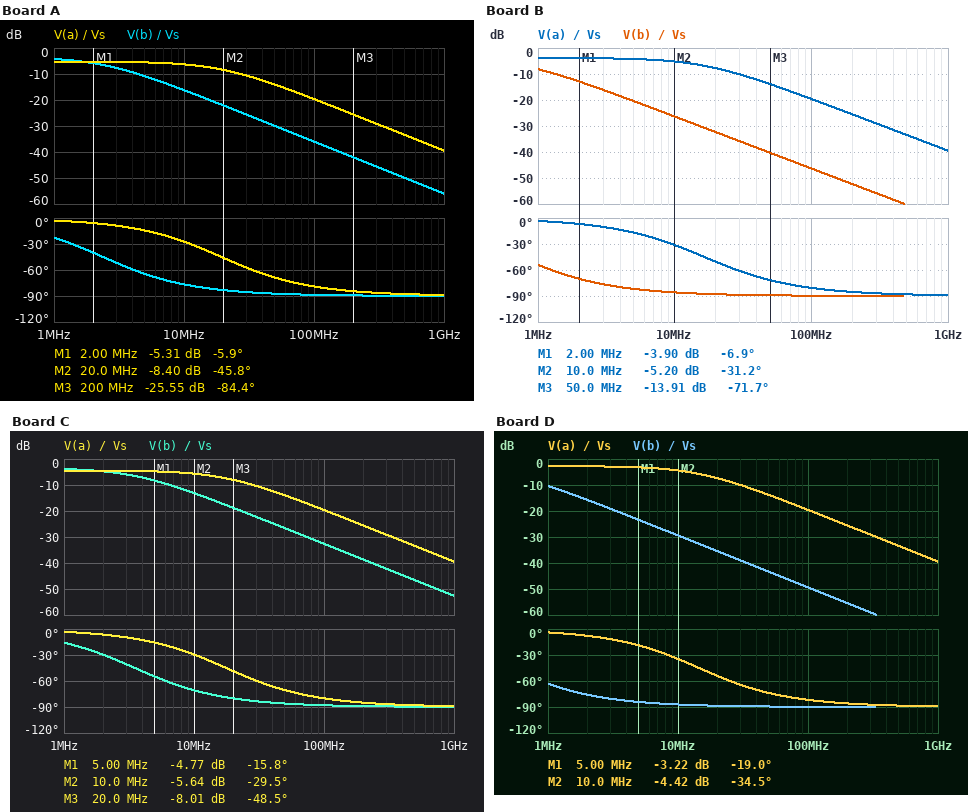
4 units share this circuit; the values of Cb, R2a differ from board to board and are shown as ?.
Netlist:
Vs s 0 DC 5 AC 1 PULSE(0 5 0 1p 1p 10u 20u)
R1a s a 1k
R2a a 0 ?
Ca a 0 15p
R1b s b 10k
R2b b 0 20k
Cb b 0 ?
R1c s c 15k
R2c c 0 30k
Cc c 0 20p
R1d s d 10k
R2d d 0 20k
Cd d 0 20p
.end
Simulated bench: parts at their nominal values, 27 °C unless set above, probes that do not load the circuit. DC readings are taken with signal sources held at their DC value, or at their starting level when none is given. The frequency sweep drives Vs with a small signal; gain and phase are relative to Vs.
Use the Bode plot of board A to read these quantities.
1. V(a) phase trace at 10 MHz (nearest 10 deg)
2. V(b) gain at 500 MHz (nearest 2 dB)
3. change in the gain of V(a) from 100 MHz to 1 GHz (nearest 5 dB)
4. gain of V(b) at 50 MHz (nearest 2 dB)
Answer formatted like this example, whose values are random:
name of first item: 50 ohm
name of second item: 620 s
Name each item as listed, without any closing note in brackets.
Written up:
V(a) phase trace at 10 MHz: -30 deg
V(b) gain at 500 MHz: -50 dB
change in the gain of V(a) from 100 MHz to 1 GHz: -20 dB
gain of V(b) at 50 MHz: -30 dB
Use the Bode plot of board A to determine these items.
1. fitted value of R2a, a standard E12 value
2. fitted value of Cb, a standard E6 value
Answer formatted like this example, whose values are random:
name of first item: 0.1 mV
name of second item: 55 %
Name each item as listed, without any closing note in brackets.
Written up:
fitted value of R2a, a standard E12 value: 1.2 kΩ
fitted value of Cb, a standard E6 value: 10 pF
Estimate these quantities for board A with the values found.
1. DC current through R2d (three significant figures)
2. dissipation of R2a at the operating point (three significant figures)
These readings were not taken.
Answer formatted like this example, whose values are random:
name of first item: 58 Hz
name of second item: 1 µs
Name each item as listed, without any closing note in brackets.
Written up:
DC current through R2d: 167 µA
dissipation of R2a at the operating point: 6.20 mW
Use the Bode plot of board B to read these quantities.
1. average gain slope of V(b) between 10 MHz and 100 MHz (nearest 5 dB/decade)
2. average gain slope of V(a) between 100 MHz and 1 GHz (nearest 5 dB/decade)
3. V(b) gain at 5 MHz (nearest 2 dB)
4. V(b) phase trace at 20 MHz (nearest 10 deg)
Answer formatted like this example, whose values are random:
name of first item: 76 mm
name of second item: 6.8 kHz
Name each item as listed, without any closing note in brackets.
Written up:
average gain slope of V(b) between 10 MHz and 100 MHz: -20 dB/decade
average gain slope of V(a) between 100 MHz and 1 GHz: -20 dB/decade
V(b) gain at 5 MHz: -20 dB
V(b) phase trace at 20 MHz: -90 deg
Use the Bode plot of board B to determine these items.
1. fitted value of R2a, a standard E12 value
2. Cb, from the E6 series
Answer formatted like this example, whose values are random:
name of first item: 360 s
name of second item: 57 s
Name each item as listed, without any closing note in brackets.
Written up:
fitted value of R2a, a standard E12 value: 1.8 kΩ
Cb, from the E6 series: 33 pF
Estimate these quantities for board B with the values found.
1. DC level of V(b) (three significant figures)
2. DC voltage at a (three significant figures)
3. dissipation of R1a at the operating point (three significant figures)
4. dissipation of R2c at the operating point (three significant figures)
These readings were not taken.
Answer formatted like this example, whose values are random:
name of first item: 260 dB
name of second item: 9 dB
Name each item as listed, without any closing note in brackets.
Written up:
DC level of V(b): 3.33 V
DC voltage at a: 3.21 V
dissipation of R1a at the operating point: 3.19 mW
dissipation of R2c at the operating point: 370 µW
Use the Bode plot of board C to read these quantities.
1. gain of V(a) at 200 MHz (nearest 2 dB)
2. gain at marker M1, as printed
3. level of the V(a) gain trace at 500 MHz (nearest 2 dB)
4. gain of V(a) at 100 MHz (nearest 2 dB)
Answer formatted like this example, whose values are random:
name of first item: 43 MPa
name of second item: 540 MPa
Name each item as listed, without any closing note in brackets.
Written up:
gain of V(a) at 200 MHz: -26 dB
gain at marker M1, as printed: -4.77 dB
level of the V(a) gain trace at 500 MHz: -34 dB
gain of V(a) at 100 MHz: -20 dB
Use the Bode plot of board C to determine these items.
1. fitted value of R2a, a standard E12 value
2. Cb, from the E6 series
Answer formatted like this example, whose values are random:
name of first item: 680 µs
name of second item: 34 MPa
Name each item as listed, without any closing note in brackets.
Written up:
fitted value of R2a, a standard E12 value: 1.5 kΩ
Cb, from the E6 series: 6.8 pF
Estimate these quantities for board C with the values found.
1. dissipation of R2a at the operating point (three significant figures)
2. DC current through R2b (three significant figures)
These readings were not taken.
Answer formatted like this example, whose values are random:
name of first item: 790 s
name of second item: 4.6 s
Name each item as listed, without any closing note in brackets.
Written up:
dissipation of R2a at the operating point: 6.00 mW
DC current through R2b: 167 µA
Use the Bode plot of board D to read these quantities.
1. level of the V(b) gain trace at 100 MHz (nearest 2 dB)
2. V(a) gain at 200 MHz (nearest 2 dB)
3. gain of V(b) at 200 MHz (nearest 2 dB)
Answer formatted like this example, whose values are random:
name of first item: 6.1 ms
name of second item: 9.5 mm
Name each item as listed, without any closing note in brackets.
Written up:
level of the V(b) gain trace at 100 MHz: -50 dB
V(a) gain at 200 MHz: -26 dB
gain of V(b) at 200 MHz: -56 dB
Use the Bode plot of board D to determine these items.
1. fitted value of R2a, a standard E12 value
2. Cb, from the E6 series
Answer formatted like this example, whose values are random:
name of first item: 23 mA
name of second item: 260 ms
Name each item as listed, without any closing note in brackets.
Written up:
fitted value of R2a, a standard E12 value: 2.7 kΩ
Cb, from the E6 series: 47 pF
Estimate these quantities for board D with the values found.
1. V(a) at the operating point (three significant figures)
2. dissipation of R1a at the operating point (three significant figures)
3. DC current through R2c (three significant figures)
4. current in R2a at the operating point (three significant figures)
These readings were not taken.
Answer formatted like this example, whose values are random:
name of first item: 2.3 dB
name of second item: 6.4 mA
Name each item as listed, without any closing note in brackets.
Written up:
V(a) at the operating point: 3.65 V
dissipation of R1a at the operating point: 1.83 mW
DC current through R2c: 111 µA
current in R2a at the operating point: 1.35 mA
